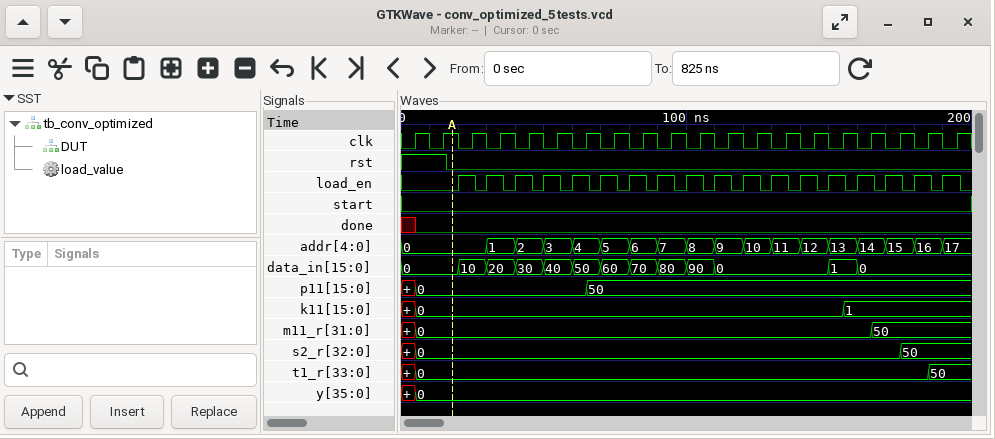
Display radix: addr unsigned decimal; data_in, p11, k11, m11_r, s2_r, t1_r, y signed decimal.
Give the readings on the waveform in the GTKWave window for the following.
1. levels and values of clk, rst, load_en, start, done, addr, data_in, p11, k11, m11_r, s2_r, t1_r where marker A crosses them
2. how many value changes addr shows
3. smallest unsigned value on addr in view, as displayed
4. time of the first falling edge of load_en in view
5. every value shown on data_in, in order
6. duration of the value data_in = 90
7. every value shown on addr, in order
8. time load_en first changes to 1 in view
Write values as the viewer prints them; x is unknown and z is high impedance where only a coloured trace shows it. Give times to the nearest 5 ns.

clk=1, rst=0, load_en=0, start=0, done=0, addr=0, data_in=0, p11=0, k11=0, m11_r=0, s2_r=0, t1_r=0
17
0
25 ns
0, 10, 20, 30, 40, 50, 60, 70, 80, 90, 0, 1, 0
10 ns
0, 1, 2, 3, 4, 5, 6, 7, 8, 9, 10, 11, 12, 13, 14, 15, 16, 17
20 ns
